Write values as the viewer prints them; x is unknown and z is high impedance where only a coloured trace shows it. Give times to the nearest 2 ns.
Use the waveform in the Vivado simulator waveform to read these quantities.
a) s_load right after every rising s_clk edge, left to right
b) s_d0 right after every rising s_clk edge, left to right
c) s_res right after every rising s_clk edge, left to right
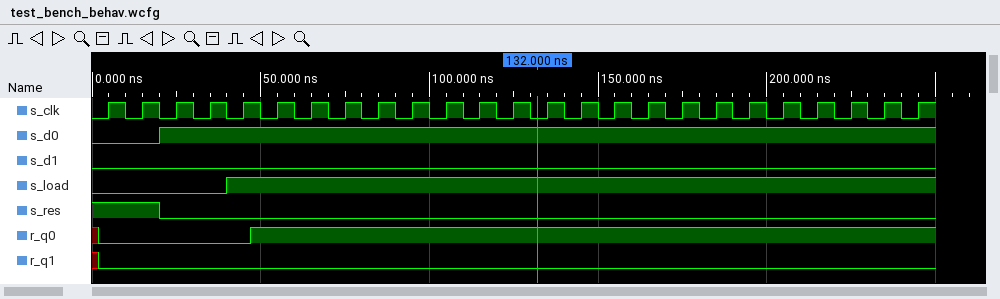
0 0 0 0 1 1 1 1 1 1 1 1 1 1 1 1 1 1 1 1 1 1 1 1 1
0 0 1 1 1 1 1 1 1 1 1 1 1 1 1 1 1 1 1 1 1 1 1 1 1
1 1 0 0 0 0 0 0 0 0 0 0 0 0 0 0 0 0 0 0 0 0 0 0 0
